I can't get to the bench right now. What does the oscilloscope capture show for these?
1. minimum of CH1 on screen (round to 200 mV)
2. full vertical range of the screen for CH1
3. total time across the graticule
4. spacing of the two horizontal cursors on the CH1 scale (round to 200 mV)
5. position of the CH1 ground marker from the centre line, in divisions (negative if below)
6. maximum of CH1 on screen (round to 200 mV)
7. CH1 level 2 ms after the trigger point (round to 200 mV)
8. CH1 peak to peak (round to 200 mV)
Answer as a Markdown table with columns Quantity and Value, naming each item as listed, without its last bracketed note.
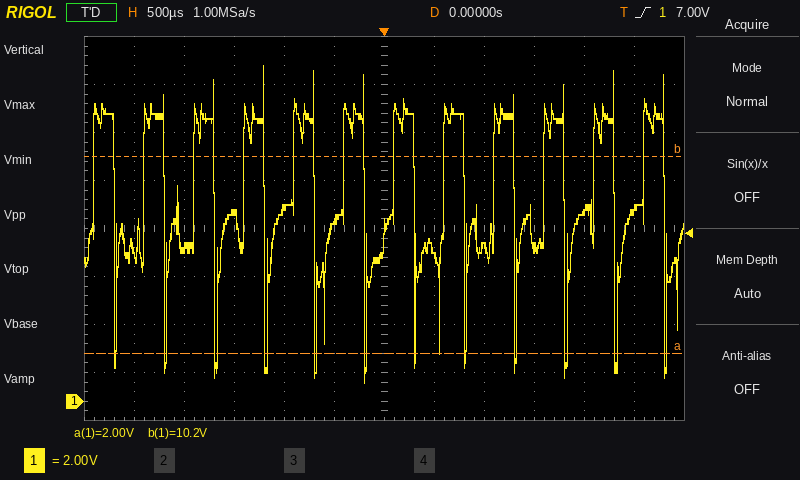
| Quantity | Value |
|---|---|
| minimum of CH1 on screen | 800 mV |
| full vertical range of the screen for CH1 | 16 V |
| total time across the graticule | 6 ms |
| spacing of the two horizontal cursors on the CH1 scale | 8.2 V |
| position of the CH1 ground marker from the centre line, in divisions | -3.6 div |
| maximum of CH1 on screen | 14.0 V |
| CH1 level 2 ms after the trigger point | 8.0 V |
| CH1 peak to peak | 13.2 V |
